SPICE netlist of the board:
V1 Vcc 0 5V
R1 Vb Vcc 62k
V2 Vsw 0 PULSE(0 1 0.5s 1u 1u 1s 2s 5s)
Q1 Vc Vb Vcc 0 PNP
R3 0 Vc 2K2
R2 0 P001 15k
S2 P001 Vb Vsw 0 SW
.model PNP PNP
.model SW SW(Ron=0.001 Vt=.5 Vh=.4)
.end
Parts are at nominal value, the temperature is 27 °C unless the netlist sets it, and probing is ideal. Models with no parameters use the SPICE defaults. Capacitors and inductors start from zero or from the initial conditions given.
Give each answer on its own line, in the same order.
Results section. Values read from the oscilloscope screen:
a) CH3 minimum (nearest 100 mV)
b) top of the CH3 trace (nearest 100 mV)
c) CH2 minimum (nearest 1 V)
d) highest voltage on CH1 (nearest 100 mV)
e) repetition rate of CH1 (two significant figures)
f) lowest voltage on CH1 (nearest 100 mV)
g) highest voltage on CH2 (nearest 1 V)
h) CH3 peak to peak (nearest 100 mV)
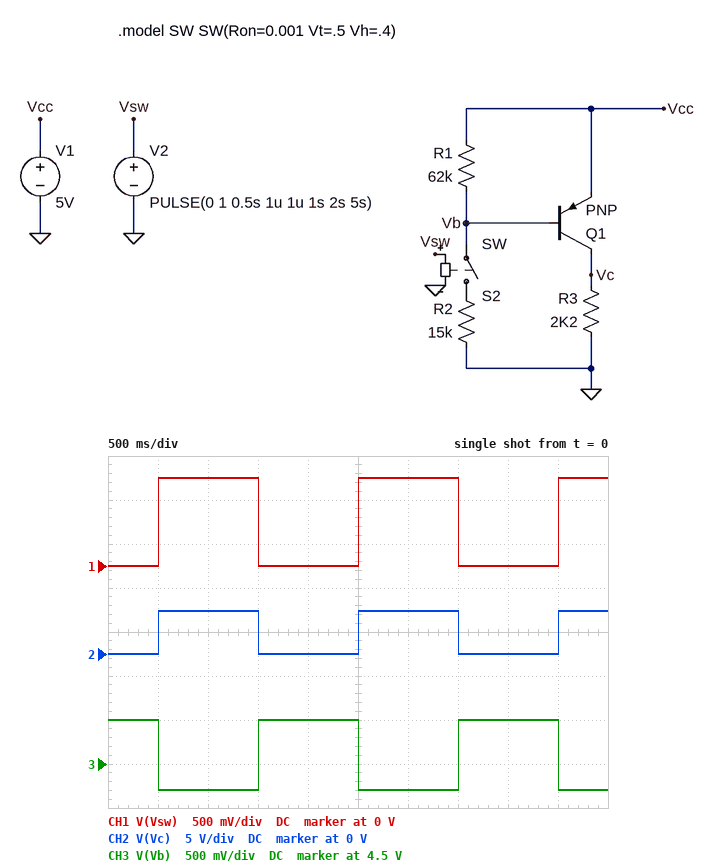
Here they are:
4.2 V
5.0 V
0 V
1.0 V
500 mHz
0 V
5 V
800 mV
